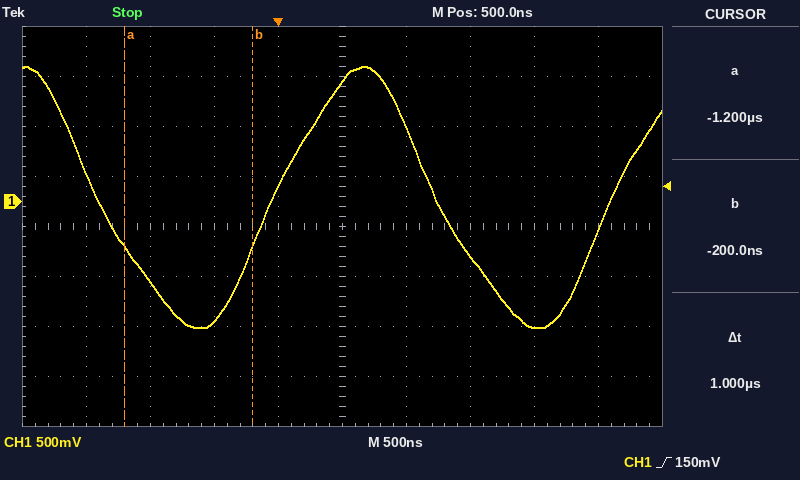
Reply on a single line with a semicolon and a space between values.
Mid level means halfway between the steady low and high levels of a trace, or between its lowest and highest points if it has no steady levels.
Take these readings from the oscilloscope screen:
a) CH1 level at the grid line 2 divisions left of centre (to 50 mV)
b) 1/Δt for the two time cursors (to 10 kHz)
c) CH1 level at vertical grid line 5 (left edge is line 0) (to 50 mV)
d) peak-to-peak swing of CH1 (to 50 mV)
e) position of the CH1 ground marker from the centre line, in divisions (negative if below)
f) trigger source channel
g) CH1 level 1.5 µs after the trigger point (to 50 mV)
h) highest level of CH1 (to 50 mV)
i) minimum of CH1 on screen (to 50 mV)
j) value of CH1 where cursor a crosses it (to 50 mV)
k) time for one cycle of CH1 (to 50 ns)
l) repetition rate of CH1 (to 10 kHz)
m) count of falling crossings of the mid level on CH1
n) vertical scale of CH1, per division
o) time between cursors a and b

-1.20 V; 1.00 MHz; 1.20 V; 2.60 V; +0.5 div; CH1; -550 mV; 1.35 V; -1.25 V; -450 mV; 2.65 µs; 380 kHz; 2; 500 mV; 1 µs
